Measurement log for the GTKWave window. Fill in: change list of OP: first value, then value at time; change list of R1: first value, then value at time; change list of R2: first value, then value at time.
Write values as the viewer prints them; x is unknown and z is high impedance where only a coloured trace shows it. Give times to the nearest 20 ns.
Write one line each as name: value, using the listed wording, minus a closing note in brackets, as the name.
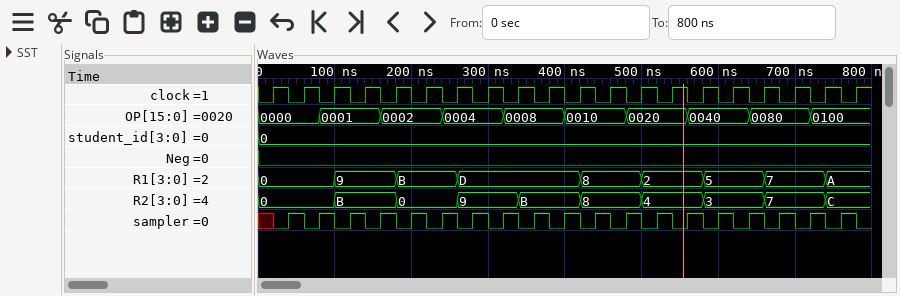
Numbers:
change list of OP: first value, then value at time: 0000, 0001 at 80 ns, 0002 at 160 ns, 0004 at 240 ns, 0008 at 320 ns, 0010 at 400 ns, 0020 at 480 ns, 0040 at 560 ns, 0080 at 640 ns, 0100 at 720 ns
change list of R1: first value, then value at time: 0, 9 at 100 ns, B at 180 ns, D at 260 ns, 8 at 420 ns, 2 at 500 ns, 5 at 580 ns, 7 at 660 ns, A at 740 ns
change list of R2: first value, then value at time: 0, B at 100 ns, 0 at 180 ns, 9 at 260 ns, B at 340 ns, 8 at 420 ns, 4 at 500 ns, 3 at 580 ns, 7 at 660 ns, C at 740 ns
